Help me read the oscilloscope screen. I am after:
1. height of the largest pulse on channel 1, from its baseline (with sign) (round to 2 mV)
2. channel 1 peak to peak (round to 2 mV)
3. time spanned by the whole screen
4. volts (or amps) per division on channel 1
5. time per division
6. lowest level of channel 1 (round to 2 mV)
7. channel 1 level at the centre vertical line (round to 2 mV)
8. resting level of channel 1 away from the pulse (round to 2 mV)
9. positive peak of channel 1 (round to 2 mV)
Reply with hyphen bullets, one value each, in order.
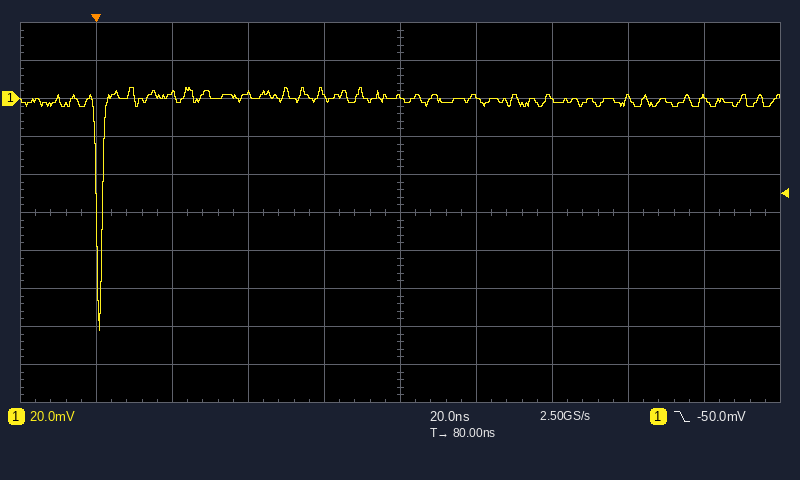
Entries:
- -122 mV
- 128 mV
- 200 ns
- 20 mV
- 20 ns
- -122 mV
- 0 mV
- 0 mV
- 6 mV
